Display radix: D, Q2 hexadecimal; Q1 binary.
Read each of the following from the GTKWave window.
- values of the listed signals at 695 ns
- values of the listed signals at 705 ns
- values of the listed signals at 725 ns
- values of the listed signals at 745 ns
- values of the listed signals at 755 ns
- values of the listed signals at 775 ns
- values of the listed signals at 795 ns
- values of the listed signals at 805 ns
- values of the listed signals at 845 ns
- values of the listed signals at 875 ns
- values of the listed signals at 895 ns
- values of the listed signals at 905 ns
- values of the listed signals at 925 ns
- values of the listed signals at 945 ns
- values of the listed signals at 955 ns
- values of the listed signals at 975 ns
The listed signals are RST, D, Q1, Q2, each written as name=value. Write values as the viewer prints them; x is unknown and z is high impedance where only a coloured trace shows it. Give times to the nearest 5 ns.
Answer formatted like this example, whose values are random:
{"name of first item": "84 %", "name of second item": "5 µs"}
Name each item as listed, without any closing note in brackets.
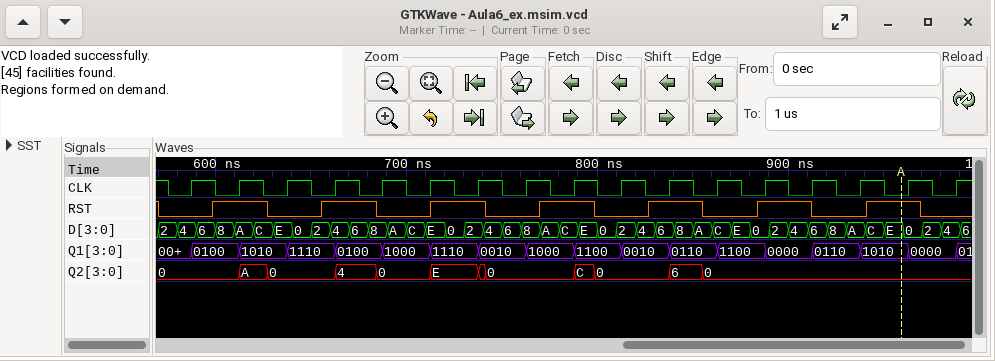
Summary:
{"values of the listed signals at 695 ns": "RST=0, D=A, Q1=1000, Q2=0", "values of the listed signals at 705 ns": "RST=0, D=C, Q1=1000, Q2=0", "values of the listed signals at 725 ns": "RST=1, D=0, Q1=1110, Q2=E", "values of the listed signals at 745 ns": "RST=0, D=4, Q1=0010, Q2=0", "values of the listed signals at 755 ns": "RST=0, D=6, Q1=0010, Q2=0", "values of the listed signals at 775 ns": "RST=1, D=A, Q1=1000, Q2=0", "values of the listed signals at 795 ns": "RST=1, D=E, Q1=1100, Q2=C", "values of the listed signals at 805 ns": "RST=0, D=0, Q1=1100, Q2=0", "values of the listed signals at 845 ns": "RST=1, D=8, Q1=0110, Q2=6", "values of the listed signals at 875 ns": "RST=0, D=E, Q1=1100, Q2=0", "values of the listed signals at 895 ns": "RST=1, D=2, Q1=0000, Q2=0", "values of the listed signals at 905 ns": "RST=1, D=4, Q1=0000, Q2=0", "values of the listed signals at 925 ns": "RST=0, D=8, Q1=0110, Q2=0", "values of the listed signals at 945 ns": "RST=1, D=C, Q1=1010, Q2=0", "values of the listed signals at 955 ns": "RST=1, D=E, Q1=1010, Q2=0", "values of the listed signals at 975 ns": "RST=0, D=2, Q1=0000, Q2=0"}
